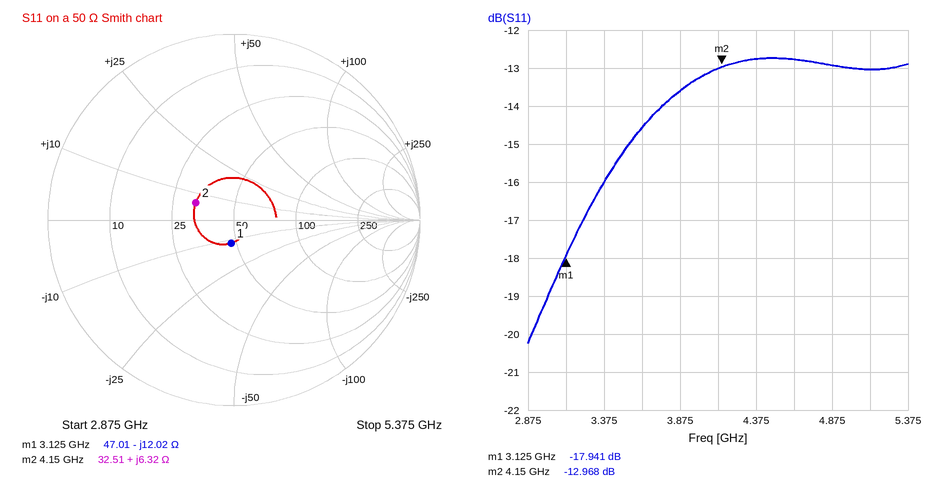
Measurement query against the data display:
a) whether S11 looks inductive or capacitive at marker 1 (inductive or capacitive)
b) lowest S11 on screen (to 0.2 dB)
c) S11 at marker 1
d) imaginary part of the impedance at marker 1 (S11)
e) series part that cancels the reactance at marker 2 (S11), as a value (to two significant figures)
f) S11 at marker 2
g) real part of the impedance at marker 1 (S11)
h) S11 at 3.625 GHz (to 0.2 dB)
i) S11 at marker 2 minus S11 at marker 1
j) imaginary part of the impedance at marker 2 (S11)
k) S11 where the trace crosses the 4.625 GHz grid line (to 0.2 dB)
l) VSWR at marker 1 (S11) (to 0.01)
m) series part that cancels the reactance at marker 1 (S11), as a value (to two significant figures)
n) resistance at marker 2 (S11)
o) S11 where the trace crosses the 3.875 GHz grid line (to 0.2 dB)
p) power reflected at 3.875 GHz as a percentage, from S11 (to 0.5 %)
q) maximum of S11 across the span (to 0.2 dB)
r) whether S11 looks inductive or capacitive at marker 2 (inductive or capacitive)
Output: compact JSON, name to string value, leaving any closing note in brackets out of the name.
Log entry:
{"whether S11 looks inductive or capacitive at marker 1": "capacitive", "lowest S11 on screen": "-20.2 dB", "S11 at marker 1": "-17.941 dB", "imaginary part of the impedance at marker 1": "-12.02 Ω", "series part that cancels the reactance at marker 2 (S11), as a value": "6.1 pF", "S11 at marker 2": "-12.968 dB", "real part of the impedance at marker 1": "47.01 Ω", "S11 at 3.625 GHz": "-14.6 dB", "S11 at marker 2 minus S11 at marker 1": "4.973 dB", "imaginary part of the impedance at marker 2": "+6.32 Ω", "S11 where the trace crosses the 4.625 GHz grid line": "-12.8 dB", "VSWR at marker 1 (S11)": "1.29", "series part that cancels the reactance at marker 1 (S11), as a value": "610 pH", "resistance at marker 2": "32.51 Ω", "S11 where the trace crosses the 3.875 GHz grid line": "-13.6 dB", "power reflected at 3.875 GHz as a percentage, from S11": "4.5 %", "maximum of S11 across the span": "-12.8 dB", "whether S11 looks inductive or capacitive at marker 2": "inductive"}
